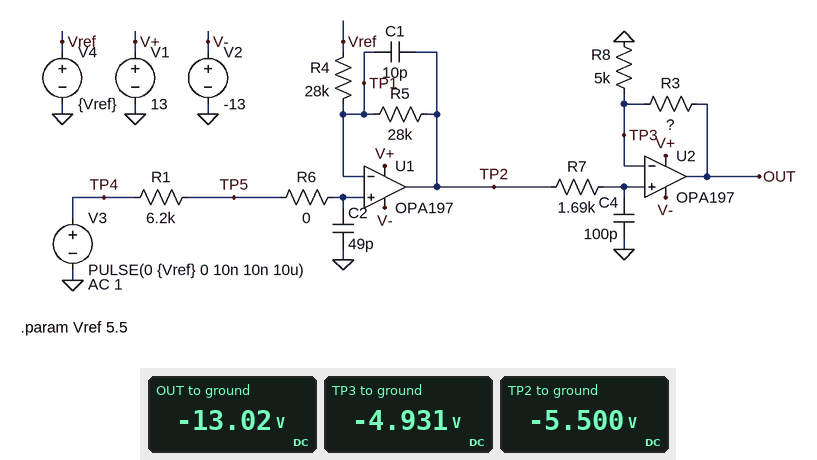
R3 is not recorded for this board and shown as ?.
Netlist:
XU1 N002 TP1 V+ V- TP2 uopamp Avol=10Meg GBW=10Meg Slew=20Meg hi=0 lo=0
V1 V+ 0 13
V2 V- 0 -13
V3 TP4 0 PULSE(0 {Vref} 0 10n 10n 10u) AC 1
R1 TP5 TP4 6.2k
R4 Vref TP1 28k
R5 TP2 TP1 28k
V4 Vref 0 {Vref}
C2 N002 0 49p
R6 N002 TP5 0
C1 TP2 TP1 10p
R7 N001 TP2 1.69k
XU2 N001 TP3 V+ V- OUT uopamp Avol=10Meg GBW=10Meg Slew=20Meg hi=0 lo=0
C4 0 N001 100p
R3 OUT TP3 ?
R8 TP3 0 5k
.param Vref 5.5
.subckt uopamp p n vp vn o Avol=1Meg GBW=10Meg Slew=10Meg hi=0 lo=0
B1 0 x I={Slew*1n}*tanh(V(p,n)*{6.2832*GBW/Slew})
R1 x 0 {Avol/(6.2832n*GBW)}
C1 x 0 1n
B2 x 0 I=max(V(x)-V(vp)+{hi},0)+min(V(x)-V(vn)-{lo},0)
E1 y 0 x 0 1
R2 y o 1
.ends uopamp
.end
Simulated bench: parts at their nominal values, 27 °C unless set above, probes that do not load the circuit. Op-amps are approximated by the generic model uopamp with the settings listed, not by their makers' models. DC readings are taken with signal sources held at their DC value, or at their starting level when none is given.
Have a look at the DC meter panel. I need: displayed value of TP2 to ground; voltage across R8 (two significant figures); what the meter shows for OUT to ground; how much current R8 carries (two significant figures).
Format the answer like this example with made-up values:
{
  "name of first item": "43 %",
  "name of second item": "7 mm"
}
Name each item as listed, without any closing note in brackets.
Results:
{
  "displayed value of TP2 to ground": "-5.500 V",
  "voltage across R8": "4.9 V",
  "what the meter shows for OUT to ground": "-13.02 V",
  "how much current R8 carries": "990 µA"
}
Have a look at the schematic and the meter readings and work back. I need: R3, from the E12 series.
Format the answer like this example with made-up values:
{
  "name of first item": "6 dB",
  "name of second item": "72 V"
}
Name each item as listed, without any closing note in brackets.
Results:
{
  "R3, from the E12 series": "8.2 kΩ"
}
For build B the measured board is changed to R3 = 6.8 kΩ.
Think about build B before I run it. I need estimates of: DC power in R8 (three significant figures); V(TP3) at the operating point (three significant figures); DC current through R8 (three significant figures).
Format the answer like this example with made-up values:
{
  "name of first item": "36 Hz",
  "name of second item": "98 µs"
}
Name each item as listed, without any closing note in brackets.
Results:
{
  "DC power in R8": "6.05 mW",
  "V(TP3) at the operating point": "-5.50 V",
  "DC current through R8": "1.10 mA"
}
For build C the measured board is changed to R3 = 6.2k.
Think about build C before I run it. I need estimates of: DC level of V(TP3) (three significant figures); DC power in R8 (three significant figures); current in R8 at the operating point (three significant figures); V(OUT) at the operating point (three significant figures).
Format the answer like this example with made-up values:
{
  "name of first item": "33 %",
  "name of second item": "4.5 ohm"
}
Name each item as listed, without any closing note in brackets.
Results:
{
  "DC level of V(TP3)": "-5.50 V",
  "DC power in R8": "6.05 mW",
  "current in R8 at the operating point": "1.10 mA",
  "V(OUT) at the operating point": "-12.3 V"
}
